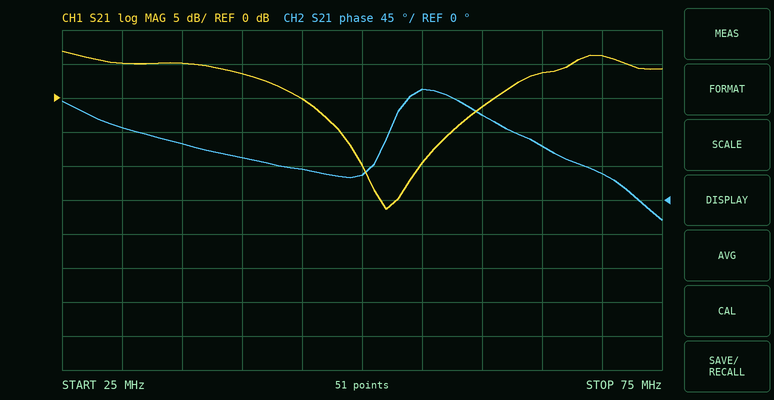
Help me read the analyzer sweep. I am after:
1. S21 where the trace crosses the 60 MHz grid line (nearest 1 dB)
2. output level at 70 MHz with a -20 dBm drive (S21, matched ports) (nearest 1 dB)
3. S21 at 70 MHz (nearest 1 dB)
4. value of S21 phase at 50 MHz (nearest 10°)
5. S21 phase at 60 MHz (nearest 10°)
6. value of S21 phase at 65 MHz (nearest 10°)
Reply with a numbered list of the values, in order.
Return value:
1. -1 dB
2. -14 dBm
3. 6 dB
4. 30°
5. 110°
6. 70°
